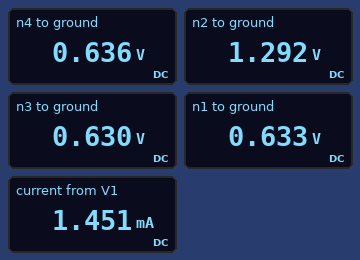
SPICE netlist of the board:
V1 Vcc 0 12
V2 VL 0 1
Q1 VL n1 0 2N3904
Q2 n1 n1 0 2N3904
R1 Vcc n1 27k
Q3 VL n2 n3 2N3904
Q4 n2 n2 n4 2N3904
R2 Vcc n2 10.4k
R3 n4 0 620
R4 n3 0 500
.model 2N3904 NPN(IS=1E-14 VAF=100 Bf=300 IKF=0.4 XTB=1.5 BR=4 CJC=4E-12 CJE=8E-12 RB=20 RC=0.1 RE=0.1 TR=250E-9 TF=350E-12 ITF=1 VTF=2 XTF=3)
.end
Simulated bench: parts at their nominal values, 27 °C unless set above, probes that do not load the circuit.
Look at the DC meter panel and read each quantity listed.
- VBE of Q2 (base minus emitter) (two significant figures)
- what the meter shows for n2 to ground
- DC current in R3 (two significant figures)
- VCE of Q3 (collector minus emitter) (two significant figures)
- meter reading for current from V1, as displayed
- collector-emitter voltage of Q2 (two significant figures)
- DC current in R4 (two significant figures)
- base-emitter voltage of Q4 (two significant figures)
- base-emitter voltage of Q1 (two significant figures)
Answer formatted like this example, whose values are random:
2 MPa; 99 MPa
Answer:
630 mV; 1.292 V; 1.0 mA; 370 mV; 1.451 mA; 630 mV; 1.3 mA; 660 mV; 630 mV
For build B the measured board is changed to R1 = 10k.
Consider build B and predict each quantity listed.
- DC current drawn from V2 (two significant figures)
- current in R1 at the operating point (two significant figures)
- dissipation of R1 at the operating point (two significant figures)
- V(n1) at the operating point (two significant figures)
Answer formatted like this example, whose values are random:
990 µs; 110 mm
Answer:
2.4 mA; 1.1 mA; 13 mW; 660 mV
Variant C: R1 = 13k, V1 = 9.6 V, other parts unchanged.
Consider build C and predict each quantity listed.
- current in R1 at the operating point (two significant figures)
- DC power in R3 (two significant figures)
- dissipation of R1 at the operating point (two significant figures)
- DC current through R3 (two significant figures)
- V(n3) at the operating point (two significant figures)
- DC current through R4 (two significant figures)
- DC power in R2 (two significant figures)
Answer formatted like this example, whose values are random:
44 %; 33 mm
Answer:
690 µA; 410 µW; 6.2 mW; 810 µA; 500 mV; 990 µA; 6.9 mW
